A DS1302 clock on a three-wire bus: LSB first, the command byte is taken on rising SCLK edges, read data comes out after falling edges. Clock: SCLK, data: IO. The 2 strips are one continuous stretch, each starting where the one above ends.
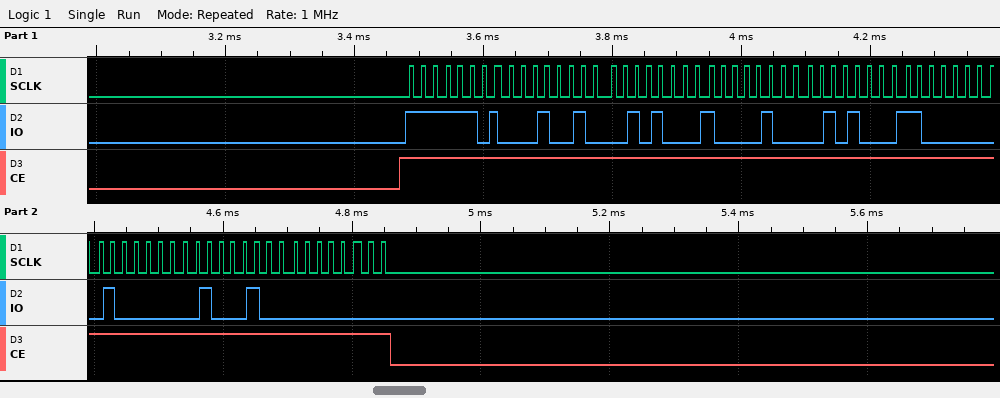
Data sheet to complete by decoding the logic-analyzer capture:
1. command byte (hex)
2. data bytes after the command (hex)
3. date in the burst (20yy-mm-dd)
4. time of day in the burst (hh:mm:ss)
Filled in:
0xBF
48 14 21 14 03 02 22 00
2022-03-14
21:14:48
